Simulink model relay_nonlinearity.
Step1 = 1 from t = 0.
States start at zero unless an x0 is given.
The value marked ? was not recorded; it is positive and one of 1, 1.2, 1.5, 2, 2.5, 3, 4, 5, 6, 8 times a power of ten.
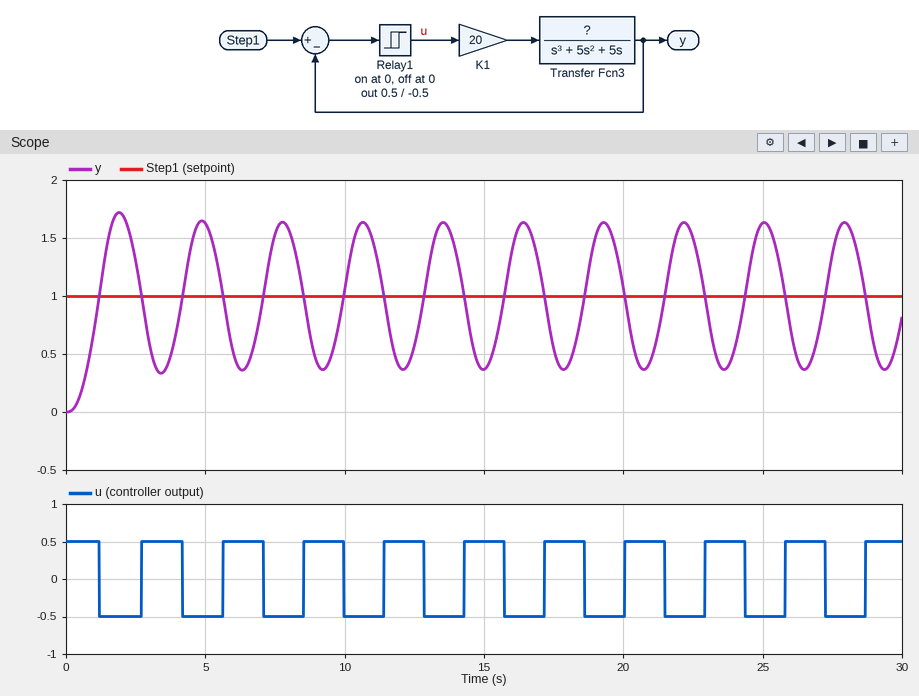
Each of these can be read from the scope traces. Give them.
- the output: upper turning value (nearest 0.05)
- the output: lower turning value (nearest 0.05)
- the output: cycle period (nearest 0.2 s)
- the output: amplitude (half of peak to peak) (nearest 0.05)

1.65
0.35
2.8 s
0.65
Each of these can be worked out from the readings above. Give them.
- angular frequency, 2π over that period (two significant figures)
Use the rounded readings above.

2.2 rad/s
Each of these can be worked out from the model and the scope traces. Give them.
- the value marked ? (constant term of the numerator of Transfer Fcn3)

1.2
